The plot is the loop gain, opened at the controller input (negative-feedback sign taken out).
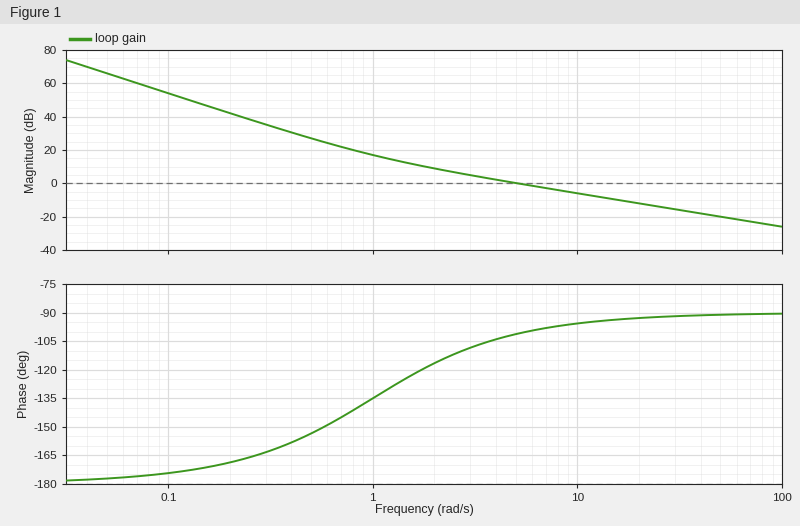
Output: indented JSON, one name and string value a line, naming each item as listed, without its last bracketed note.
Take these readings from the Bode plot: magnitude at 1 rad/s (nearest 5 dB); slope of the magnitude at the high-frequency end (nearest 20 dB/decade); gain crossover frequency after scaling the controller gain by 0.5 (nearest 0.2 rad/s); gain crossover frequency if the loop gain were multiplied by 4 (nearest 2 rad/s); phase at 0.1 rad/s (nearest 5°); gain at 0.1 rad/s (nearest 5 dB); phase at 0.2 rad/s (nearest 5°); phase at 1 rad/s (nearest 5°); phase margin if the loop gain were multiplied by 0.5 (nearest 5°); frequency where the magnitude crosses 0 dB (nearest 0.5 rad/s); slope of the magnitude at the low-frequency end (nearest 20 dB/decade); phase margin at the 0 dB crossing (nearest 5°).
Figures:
{
  "magnitude at 1 rad/s": "15 dB",
  "slope of the magnitude at the high-frequency end": "-20 dB/decade",
  "gain crossover frequency after scaling the controller gain by 0.5": "2.6 rad/s",
  "gain crossover frequency if the loop gain were multiplied by 4": "20 rad/s",
  "phase at 0.1 rad/s": "-175°",
  "gain at 0.1 rad/s": "55 dB",
  "phase at 0.2 rad/s": "-170°",
  "phase at 1 rad/s": "-135°",
  "phase margin if the loop gain were multiplied by 0.5": "70°",
  "frequency where the magnitude crosses 0 dB": "5.0 rad/s",
  "slope of the magnitude at the low-frequency end": "-40 dB/decade",
  "phase margin at the 0 dB crossing": "80°"
}
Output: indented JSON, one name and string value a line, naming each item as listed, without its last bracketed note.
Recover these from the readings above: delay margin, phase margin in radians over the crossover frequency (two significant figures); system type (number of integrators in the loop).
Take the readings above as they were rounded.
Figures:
{
  "delay margin, phase margin in radians over the crossover frequency": "0.28 s",
  "system type": "2"
}
